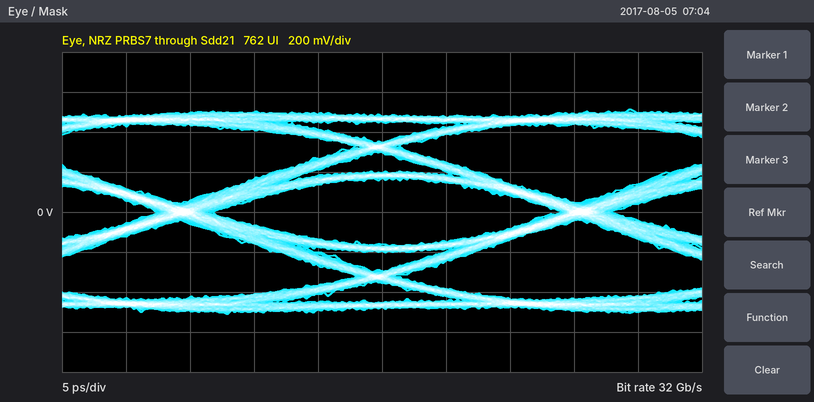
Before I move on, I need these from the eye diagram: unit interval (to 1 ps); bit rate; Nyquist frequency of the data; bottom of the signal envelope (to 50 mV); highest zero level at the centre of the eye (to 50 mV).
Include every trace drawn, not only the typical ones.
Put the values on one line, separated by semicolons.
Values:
31 ps; 32 Gb/s; 16 GHz; -500 mV; -150 mV
